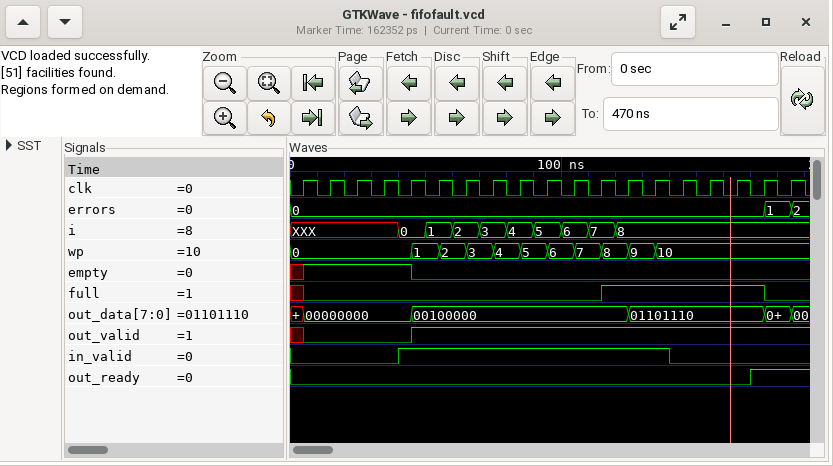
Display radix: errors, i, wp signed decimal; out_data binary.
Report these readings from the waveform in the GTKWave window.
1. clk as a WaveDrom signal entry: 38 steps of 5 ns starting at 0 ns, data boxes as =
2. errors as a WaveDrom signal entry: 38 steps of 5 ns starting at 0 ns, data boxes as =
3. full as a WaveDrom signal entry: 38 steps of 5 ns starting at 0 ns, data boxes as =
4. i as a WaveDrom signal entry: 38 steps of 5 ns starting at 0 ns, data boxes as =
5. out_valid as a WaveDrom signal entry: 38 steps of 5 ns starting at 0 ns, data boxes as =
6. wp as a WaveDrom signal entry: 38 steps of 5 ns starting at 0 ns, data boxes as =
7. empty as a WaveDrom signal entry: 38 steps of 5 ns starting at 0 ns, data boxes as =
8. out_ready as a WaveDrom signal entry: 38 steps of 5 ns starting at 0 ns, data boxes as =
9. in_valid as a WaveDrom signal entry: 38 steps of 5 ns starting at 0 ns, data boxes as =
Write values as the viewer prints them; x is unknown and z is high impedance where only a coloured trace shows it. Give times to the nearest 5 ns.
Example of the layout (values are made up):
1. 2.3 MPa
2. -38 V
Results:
1. {name: 'clk', wave: '01010101010101010101010101010101010101'}
2. {name: 'errors', wave: '=..................................=.=', data: '0 1 2'}
3. {name: 'full', wave: 'x0.....................1...........0..'}
4. {name: 'i', wave: 'x.......=.=.=.=.=.=.=.=.=.............', data: '0 1 2 3 4 5 6 7 8'}
5. {name: 'out_valid', wave: 'x0.......1............................'}
6. {name: 'wp', wave: '=........=.=.=.=.=.=.=.=.=.=..........', data: '0 1 2 3 4 5 6 7 8 9 10'}
7. {name: 'empty', wave: 'x1.......0............................'}
8. {name: 'out_ready', wave: '0.................................1...'}
9. {name: 'in_valid', wave: '0.......1...................0.........'}
